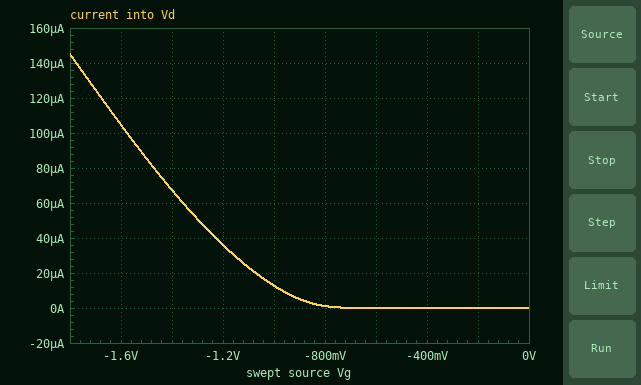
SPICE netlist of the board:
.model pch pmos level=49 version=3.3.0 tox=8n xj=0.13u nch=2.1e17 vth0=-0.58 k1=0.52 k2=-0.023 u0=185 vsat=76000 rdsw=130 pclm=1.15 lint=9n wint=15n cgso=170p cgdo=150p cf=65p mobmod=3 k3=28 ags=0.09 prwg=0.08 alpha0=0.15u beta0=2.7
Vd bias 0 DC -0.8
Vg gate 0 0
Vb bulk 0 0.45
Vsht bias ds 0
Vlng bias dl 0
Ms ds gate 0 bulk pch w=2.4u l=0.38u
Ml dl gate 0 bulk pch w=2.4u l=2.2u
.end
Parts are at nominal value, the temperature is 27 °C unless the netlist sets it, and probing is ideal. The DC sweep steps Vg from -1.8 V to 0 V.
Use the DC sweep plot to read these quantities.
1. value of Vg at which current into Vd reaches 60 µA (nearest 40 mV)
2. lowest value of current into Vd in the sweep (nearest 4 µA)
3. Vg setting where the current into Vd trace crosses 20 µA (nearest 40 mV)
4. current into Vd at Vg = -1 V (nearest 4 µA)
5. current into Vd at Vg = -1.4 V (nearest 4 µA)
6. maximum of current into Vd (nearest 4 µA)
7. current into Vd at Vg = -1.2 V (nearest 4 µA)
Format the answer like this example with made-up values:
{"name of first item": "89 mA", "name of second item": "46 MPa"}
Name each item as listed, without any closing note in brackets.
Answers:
{"value of Vg at which current into Vd reaches 60 µA": "-1.36 V", "lowest value of current into Vd in the sweep": "0 A", "Vg setting where the current into Vd trace crosses 20 µA": "-1.08 V", "current into Vd at Vg = -1 V": "12 µA", "current into Vd at Vg = -1.4 V": "68 µA", "maximum of current into Vd": "144 µA", "current into Vd at Vg = -1.2 V": "36 µA"}
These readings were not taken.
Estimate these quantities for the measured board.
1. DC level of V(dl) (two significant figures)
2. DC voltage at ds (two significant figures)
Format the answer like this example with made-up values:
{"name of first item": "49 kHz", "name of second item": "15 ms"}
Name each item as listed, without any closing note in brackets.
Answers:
{"DC level of V(dl)": "-800 mV", "DC voltage at ds": "-800 mV"}
